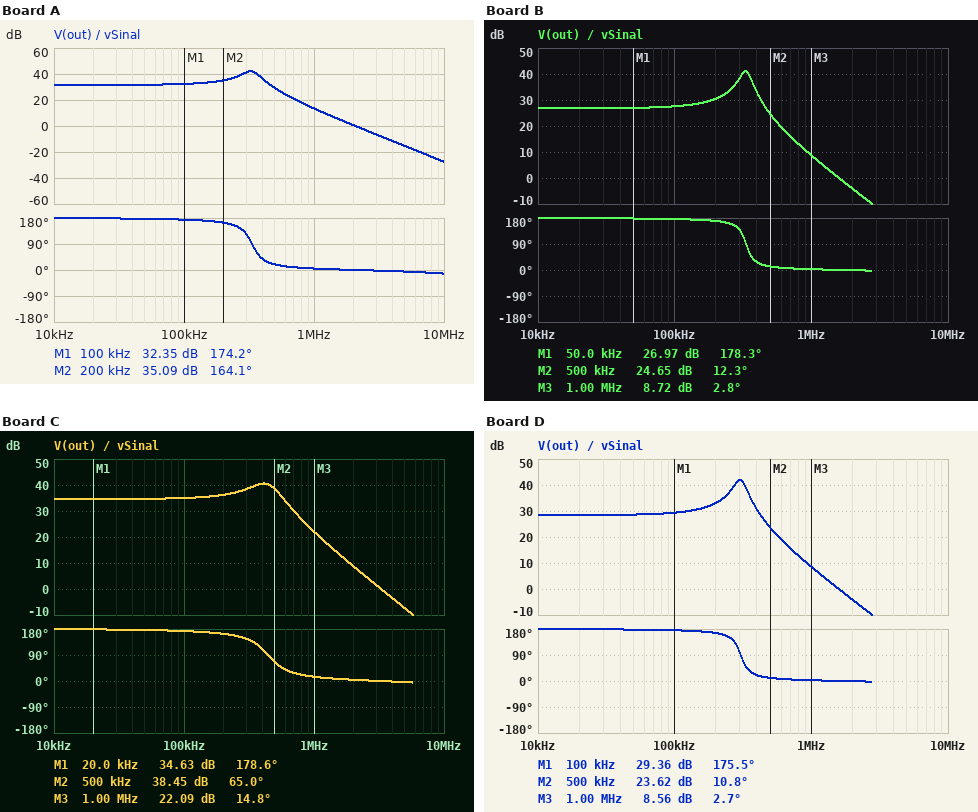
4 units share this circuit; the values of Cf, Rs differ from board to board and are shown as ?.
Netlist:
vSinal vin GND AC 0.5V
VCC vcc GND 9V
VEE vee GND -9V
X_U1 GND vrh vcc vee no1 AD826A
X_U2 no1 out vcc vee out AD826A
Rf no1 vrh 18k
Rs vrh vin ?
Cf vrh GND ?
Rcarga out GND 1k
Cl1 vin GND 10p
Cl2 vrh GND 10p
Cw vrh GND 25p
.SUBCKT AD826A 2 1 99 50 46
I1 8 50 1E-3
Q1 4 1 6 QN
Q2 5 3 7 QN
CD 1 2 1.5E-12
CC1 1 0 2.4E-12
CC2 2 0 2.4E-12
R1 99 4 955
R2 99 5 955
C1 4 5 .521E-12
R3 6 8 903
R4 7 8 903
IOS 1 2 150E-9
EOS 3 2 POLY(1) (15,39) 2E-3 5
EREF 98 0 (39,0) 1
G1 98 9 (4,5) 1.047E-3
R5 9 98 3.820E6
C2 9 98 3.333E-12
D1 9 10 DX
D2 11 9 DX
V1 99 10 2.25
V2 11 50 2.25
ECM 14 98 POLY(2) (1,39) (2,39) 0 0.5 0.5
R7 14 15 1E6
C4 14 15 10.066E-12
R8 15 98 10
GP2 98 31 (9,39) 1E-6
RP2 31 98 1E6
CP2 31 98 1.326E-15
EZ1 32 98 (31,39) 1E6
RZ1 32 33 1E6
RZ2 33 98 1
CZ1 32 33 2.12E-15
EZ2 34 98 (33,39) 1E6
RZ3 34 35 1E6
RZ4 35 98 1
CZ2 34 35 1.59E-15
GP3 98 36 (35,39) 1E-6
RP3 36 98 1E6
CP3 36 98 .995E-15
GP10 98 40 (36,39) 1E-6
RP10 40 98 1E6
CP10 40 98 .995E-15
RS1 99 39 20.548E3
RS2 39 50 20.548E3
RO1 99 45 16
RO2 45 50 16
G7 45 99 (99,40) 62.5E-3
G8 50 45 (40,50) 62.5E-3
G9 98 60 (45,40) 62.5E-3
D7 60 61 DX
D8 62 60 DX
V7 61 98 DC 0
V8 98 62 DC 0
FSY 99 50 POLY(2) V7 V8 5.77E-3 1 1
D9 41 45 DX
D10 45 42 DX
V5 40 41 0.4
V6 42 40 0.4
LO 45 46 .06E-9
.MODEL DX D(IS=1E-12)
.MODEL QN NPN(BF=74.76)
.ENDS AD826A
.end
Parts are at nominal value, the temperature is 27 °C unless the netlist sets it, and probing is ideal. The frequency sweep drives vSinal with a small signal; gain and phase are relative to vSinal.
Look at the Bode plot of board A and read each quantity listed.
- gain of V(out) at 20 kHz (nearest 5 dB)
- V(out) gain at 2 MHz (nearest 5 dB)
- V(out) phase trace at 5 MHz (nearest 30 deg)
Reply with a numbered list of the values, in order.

1. 30 dB
2. 0 dB
3. 0 deg
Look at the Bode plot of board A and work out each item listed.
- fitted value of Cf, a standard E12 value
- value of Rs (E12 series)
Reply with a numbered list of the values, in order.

1. 3.9 nF
2. 470 Ω
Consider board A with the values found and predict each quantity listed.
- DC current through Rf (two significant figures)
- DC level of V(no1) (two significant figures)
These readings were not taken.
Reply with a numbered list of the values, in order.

1. 11 µA
2. 200 mV
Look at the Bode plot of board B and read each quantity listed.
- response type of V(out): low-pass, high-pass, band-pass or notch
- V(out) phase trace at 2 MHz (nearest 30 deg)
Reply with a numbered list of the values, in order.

1. low-pass
2. 0 deg
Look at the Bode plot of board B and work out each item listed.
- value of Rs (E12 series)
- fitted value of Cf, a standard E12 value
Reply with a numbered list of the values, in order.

1. 820 Ω
2. 3.9 nF
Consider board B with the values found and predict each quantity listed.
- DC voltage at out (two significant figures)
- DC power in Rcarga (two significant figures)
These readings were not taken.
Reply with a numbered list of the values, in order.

1. 170 mV
2. 28 µW
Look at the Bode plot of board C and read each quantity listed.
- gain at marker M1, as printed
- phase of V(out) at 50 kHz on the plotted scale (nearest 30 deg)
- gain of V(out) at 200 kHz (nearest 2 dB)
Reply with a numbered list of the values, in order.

1. 34.63 dB
2. 180 deg
3. 36 dB
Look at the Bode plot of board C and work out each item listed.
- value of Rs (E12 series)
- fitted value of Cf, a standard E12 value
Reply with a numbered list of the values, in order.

1. 330 Ω
2. 2.2 nF
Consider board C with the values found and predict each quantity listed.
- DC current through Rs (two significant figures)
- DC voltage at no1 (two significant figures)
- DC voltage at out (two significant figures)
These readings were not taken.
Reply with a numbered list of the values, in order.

1. 5.9 µA
2. 230 mV
3. 230 mV
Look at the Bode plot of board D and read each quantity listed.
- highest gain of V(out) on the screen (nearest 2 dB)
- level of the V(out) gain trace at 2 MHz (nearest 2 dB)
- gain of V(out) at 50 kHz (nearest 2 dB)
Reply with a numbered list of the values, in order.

1. 42 dB
2. -4 dB
3. 28 dB
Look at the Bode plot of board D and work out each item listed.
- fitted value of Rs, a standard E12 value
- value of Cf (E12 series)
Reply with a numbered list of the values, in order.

1. 680 Ω
2. 4.7 nF
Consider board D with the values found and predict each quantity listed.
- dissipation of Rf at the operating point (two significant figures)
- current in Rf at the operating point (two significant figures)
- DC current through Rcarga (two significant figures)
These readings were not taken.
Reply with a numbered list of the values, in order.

1. 1.7 µW
2. 9.6 µA
3. 180 µA
